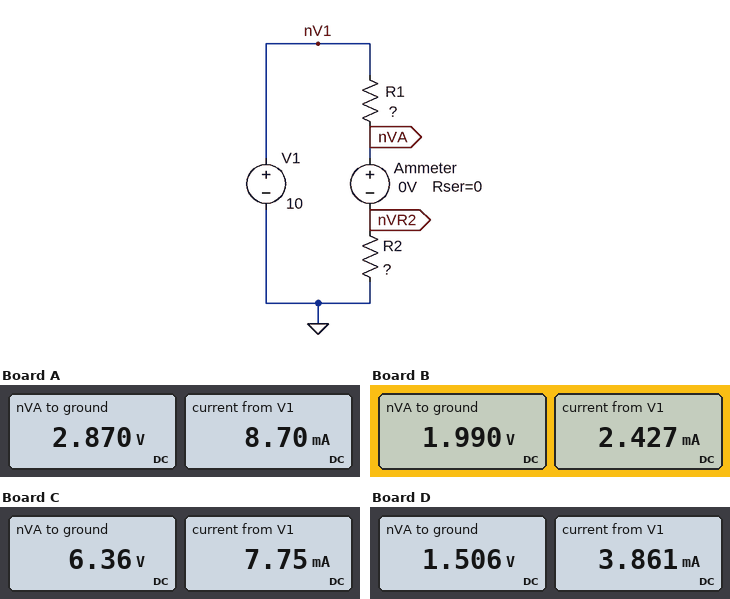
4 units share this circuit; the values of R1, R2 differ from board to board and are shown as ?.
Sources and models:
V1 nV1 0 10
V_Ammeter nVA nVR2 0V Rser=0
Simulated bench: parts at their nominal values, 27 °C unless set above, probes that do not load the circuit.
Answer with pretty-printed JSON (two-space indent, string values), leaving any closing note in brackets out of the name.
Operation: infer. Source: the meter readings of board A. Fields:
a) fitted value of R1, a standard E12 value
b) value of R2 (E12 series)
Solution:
{
  "fitted value of R1, a standard E12 value": "820 Ω",
  "value of R2": "330 Ω"
}
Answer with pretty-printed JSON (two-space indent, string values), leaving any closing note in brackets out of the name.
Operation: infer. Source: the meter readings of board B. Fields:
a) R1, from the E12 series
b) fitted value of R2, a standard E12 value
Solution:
{
  "R1, from the E12 series": "3.3 kΩ",
  "fitted value of R2, a standard E12 value": "820 Ω"
}
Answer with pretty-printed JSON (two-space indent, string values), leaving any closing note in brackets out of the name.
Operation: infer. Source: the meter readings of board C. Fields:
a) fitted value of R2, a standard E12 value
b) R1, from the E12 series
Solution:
{
  "fitted value of R2, a standard E12 value": "820 Ω",
  "R1, from the E12 series": "470 Ω"
}
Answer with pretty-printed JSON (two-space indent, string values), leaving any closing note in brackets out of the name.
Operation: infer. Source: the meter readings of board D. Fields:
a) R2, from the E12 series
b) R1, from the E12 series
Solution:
{
  "R2, from the E12 series": "390 Ω",
  "R1, from the E12 series": "2.2 kΩ"
}
